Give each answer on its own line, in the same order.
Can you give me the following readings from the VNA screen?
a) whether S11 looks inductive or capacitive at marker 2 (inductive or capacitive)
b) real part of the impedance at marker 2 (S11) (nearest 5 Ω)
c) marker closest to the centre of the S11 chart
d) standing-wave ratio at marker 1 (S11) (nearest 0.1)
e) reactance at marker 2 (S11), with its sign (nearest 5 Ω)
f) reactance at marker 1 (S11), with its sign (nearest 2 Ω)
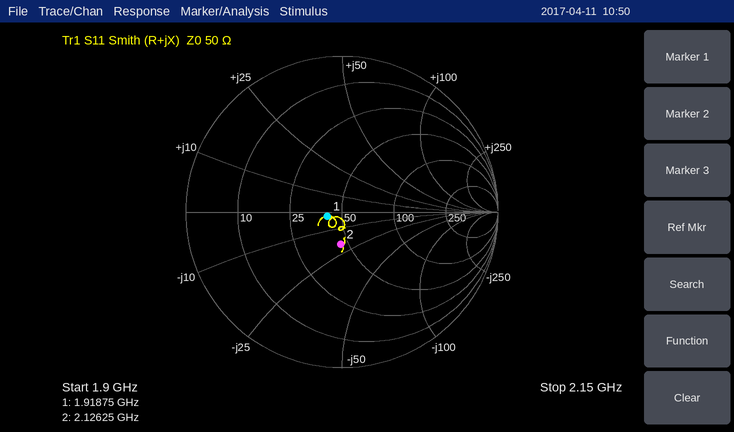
capacitive
45 Ω
marker 1
1.2
-20 Ω
-2 Ω
